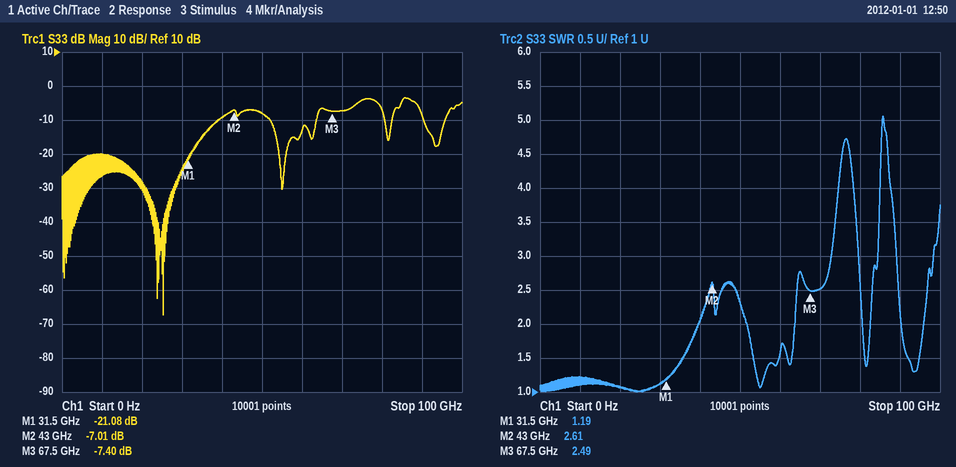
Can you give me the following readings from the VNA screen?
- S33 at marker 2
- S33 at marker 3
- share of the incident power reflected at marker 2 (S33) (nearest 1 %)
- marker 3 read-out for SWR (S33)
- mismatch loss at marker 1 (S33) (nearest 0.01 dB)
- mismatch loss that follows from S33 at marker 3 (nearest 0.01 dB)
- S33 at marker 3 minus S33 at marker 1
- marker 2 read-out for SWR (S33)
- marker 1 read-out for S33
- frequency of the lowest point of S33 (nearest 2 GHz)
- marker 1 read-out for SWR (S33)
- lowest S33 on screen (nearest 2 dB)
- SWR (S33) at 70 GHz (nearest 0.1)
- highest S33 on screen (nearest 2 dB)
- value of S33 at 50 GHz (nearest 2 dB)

-7.01 dB
-7.40 dB
20 %
2.49
0.03 dB
0.87 dB
13.68 dB
2.61
-21.08 dB
26 GHz
1.19
-68 dB
2.5
-4 dB
-8 dB
